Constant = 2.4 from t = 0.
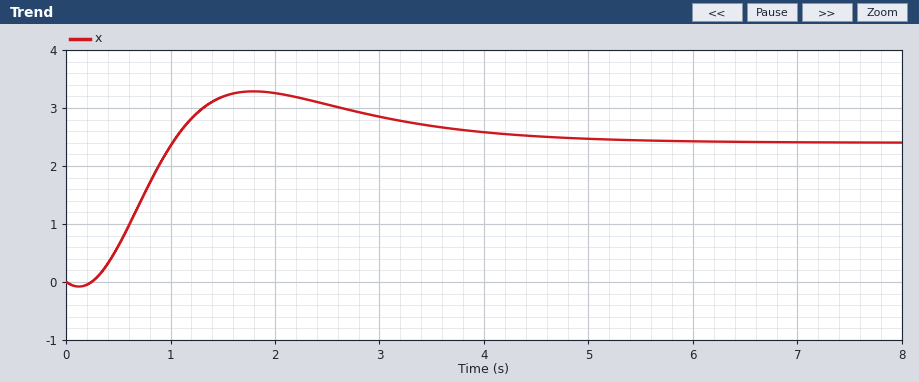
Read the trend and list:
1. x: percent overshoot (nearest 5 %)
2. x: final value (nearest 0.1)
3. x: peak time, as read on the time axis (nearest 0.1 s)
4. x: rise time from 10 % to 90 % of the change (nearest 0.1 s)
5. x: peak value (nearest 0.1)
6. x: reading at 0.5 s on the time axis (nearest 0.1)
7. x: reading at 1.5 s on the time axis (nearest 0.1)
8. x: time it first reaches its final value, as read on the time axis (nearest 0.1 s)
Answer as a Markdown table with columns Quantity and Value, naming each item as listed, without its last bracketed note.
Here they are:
| Quantity | Value |
|---|---|
| x: percent overshoot | 35 % |
| x: final value | 2.4 |
| x: peak time, as read on the time axis | 1.8 s |
| x: rise time from 10 % to 90 % of the change | 0.6 s |
| x: peak value | 3.3 |
| x: reading at 0.5 s on the time axis | 0.6 |
| x: reading at 1.5 s on the time axis | 3.2 |
| x: time it first reaches its final value, as read on the time axis | 1.0 s |
